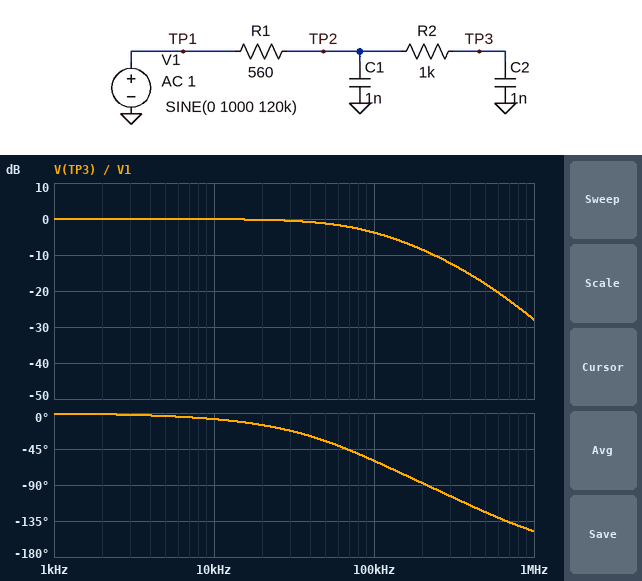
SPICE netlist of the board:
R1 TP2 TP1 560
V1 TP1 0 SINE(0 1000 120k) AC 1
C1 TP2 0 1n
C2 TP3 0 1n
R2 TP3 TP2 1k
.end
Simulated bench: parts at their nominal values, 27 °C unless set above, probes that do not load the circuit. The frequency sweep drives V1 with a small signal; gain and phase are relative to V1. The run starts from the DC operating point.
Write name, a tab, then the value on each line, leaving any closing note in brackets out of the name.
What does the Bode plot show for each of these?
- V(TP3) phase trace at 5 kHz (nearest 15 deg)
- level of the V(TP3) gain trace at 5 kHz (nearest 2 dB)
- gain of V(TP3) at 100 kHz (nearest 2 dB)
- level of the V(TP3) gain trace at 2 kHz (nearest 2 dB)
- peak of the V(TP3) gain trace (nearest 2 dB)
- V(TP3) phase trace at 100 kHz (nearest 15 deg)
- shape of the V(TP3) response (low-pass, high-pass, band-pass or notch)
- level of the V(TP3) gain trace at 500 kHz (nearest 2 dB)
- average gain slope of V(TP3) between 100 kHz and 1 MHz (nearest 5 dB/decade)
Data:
V(TP3) phase trace at 5 kHz	0 deg
level of the V(TP3) gain trace at 5 kHz	0 dB
gain of V(TP3) at 100 kHz	-4 dB
level of the V(TP3) gain trace at 2 kHz	0 dB
peak of the V(TP3) gain trace	0 dB
V(TP3) phase trace at 100 kHz	-60 deg
shape of the V(TP3) response	low-pass
level of the V(TP3) gain trace at 500 kHz	-18 dB
average gain slope of V(TP3) between 100 kHz and 1 MHz	-25 dB/decade
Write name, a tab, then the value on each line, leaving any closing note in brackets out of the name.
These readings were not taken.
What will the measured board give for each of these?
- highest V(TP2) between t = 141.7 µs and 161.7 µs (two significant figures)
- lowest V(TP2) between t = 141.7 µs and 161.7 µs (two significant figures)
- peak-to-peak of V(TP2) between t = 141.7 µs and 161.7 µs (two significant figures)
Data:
highest V(TP2) between t = 141.7 µs and 161.7 µs	720 V
lowest V(TP2) between t = 141.7 µs and 161.7 µs	-720 V
peak-to-peak of V(TP2) between t = 141.7 µs and 161.7 µs	1.4 kV
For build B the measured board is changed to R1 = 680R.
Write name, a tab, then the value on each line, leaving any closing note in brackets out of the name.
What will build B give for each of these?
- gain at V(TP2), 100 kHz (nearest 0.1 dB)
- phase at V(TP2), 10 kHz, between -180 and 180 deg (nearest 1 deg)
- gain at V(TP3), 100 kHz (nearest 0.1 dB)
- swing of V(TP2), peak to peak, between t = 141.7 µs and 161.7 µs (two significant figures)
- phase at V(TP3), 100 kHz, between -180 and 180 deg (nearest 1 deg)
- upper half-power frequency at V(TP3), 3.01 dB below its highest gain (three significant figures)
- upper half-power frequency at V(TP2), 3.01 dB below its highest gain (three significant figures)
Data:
gain at V(TP2), 100 kHz	-2.9 dB
phase at V(TP2), 10 kHz, between -180 and 180 deg	-5 deg
gain at V(TP3), 100 kHz	-4.4 dB
swing of V(TP2), peak to peak, between t = 141.7 µs and 161.7 µs	1.3 kV
phase at V(TP3), 100 kHz, between -180 and 180 deg	-64 deg
upper half-power frequency at V(TP3), 3.01 dB below its highest gain	76.6 kHz
upper half-power frequency at V(TP2), 3.01 dB below its highest gain	103 kHz
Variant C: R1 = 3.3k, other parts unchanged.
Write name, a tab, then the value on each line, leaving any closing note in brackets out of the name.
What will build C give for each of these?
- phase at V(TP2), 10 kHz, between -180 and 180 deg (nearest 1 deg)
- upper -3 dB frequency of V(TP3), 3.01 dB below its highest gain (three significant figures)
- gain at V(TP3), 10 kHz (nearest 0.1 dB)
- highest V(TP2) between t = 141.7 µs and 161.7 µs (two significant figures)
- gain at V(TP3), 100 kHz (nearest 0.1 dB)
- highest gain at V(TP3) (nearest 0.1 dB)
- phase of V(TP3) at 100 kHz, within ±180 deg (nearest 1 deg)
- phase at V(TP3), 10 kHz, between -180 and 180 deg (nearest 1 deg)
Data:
phase at V(TP2), 10 kHz, between -180 and 180 deg	-22 deg
upper -3 dB frequency of V(TP3), 3.01 dB below its highest gain	22.2 kHz
gain at V(TP3), 10 kHz	-0.8 dB
highest V(TP2) between t = 141.7 µs and 161.7 µs	220 V
gain at V(TP3), 100 kHz	-13.6 dB
highest gain at V(TP3)	0 dB
phase of V(TP3) at 100 kHz, within ±180 deg	-94 deg
phase at V(TP3), 10 kHz, between -180 and 180 deg	-26 deg
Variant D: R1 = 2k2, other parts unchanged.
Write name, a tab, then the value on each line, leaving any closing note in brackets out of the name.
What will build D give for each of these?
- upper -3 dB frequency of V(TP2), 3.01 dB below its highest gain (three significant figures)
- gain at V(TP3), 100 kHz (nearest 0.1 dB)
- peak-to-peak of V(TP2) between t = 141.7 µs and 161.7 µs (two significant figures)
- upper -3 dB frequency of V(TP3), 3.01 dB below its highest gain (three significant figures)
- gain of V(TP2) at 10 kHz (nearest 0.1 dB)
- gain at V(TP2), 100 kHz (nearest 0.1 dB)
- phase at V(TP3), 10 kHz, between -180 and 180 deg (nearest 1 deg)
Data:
upper -3 dB frequency of V(TP2), 3.01 dB below its highest gain	33.2 kHz
gain at V(TP3), 100 kHz	-10.6 dB
peak-to-peak of V(TP2) between t = 141.7 µs and 161.7 µs	610 V
upper -3 dB frequency of V(TP3), 3.01 dB below its highest gain	31.9 kHz
gain of V(TP2) at 10 kHz	-0.4 dB
gain at V(TP2), 100 kHz	-9.2 dB
phase at V(TP3), 10 kHz, between -180 and 180 deg	-19 deg
